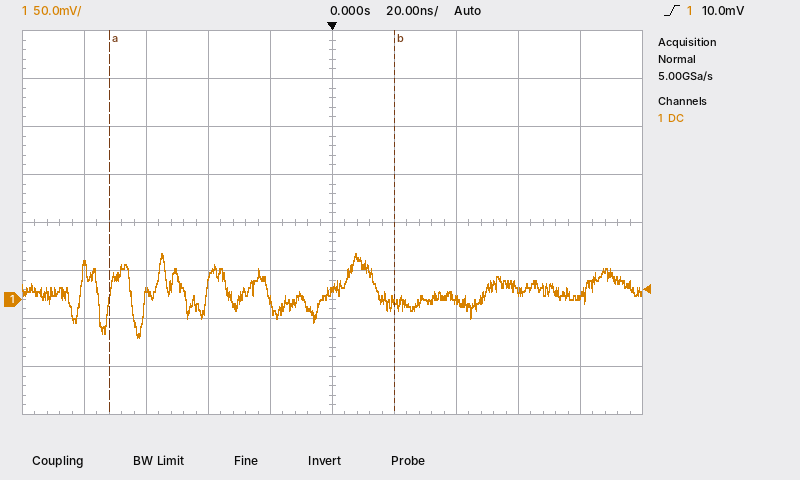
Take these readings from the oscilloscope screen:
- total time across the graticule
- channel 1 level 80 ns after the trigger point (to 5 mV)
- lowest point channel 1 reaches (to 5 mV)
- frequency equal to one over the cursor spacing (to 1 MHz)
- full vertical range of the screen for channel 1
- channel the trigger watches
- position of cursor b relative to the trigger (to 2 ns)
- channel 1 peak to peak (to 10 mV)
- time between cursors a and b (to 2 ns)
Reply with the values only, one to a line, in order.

200 ns
5 mV
-40 mV
11 MHz
400 mV
channel 1
+20 ns
90 mV
92 ns
